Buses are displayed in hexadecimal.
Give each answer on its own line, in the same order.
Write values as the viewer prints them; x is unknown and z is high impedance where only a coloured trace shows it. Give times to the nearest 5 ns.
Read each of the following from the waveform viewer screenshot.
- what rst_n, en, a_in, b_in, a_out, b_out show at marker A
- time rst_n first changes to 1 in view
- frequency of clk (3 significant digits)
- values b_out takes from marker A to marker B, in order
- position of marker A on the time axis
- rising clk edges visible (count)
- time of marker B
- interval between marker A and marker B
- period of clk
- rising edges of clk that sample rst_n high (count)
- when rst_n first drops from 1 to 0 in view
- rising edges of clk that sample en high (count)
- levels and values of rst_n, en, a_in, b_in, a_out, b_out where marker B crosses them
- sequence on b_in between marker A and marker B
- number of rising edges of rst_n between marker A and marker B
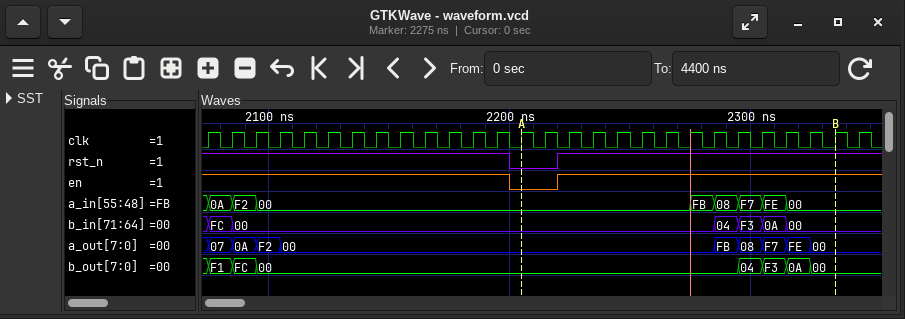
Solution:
rst_n=0, en=0, a_in=00, b_in=00, a_out=00, b_out=00
2220 ns
100 MHz
00, 04, F3, 0A, 00
2205 ns
28
2335 ns
130 ns
10 ns
26
2200 ns
26
rst_n=1, en=1, a_in=00, b_in=00, a_out=00, b_out=00
00, 04, F3, 0A, 00
1
